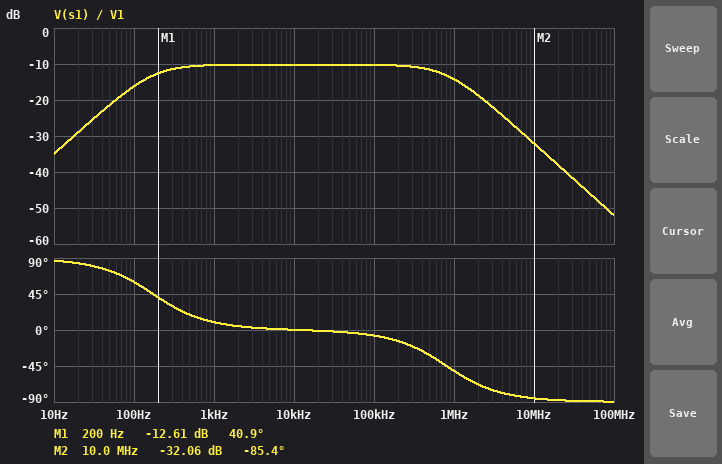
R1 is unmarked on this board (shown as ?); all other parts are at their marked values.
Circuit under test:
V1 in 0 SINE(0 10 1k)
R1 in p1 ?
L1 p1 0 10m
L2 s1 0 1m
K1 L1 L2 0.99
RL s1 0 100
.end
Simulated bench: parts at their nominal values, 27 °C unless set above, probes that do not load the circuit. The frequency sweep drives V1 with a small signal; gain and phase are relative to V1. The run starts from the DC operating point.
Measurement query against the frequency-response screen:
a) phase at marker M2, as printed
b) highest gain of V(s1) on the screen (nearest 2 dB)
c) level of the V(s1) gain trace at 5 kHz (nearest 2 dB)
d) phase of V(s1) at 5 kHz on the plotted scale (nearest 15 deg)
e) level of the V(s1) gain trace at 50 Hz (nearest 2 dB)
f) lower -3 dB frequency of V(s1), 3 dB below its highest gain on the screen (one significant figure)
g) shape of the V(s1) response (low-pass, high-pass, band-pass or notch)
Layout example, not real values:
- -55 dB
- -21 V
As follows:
- -85.4 deg
- -10 dB
- -10 dB
- 0 deg
- -22 dB
- 200 Hz
- band-pass
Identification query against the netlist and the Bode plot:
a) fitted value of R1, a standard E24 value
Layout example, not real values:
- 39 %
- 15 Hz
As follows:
- 11 Ω
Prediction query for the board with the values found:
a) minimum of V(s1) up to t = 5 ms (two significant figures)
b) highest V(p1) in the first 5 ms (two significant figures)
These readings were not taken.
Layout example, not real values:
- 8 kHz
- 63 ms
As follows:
- -3.3 V
- 9.7 V
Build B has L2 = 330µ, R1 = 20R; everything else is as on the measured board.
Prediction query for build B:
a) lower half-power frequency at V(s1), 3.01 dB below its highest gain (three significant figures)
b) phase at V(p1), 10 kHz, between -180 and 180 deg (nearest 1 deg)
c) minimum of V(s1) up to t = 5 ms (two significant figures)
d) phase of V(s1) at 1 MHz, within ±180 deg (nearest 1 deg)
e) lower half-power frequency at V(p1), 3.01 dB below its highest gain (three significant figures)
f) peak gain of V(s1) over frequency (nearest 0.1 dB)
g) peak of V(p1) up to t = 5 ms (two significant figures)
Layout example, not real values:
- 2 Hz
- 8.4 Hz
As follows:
- 316 Hz
- 2 deg
- -1.8 V
- -22 deg
- 320 Hz
- -15.0 dB
- 9.5 V
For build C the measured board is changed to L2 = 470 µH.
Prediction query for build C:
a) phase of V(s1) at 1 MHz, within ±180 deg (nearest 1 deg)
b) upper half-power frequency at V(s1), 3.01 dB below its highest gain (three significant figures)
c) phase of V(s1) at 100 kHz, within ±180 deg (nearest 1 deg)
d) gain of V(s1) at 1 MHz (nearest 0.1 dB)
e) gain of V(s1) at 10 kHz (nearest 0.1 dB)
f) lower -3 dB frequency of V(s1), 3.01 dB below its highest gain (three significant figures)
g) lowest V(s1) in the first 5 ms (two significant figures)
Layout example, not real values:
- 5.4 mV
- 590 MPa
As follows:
- -30 deg
- 1.71 MHz
- -3 deg
- -14.7 dB
- -13.4 dB
- 174 Hz
- -2.3 V
